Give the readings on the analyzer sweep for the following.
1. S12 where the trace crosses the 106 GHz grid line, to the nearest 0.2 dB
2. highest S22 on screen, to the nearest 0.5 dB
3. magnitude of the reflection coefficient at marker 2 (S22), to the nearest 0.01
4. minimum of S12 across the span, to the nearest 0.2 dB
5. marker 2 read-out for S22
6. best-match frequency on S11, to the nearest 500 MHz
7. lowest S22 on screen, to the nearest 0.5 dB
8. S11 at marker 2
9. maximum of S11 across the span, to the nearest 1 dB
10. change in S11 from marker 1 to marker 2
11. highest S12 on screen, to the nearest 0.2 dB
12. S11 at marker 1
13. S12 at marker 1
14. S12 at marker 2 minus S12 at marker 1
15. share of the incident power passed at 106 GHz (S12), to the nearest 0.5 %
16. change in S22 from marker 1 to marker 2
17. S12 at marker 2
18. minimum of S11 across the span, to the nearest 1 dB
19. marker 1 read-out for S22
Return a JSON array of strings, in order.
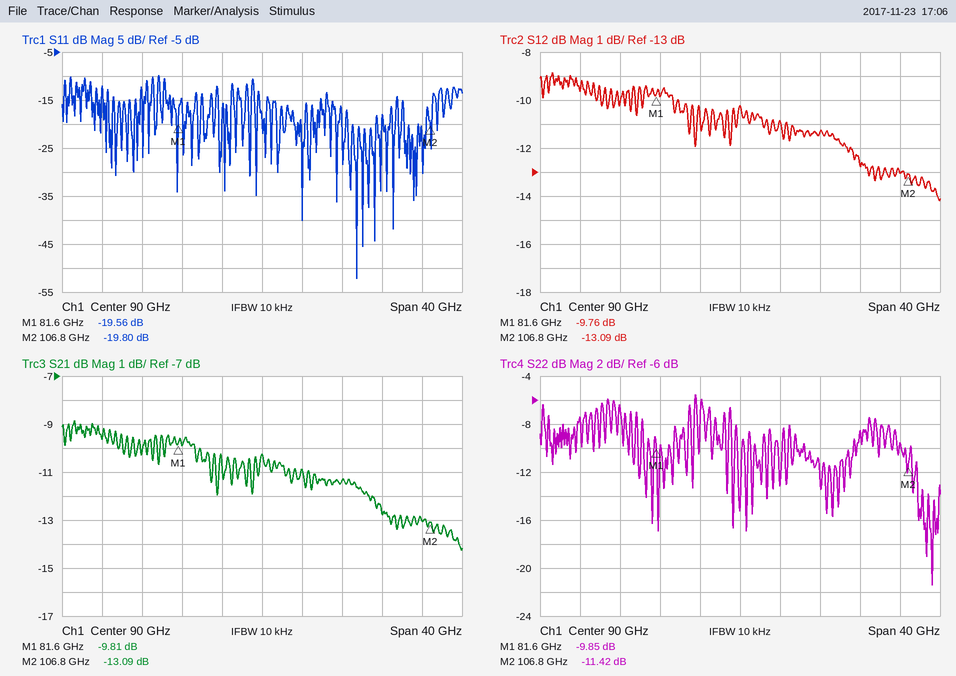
["-13.0 dB", "-5.5 dB", "0.27", "-14.2 dB", "-11.42 dB", "99.5 GHz", "-21.5 dB", "-19.80 dB", "-10 dB", "-0.24 dB", "-8.8 dB", "-19.56 dB", "-9.76 dB", "-3.33 dB", "5.0 %", "-1.57 dB", "-13.09 dB", "-52 dB", "-9.85 dB"]
